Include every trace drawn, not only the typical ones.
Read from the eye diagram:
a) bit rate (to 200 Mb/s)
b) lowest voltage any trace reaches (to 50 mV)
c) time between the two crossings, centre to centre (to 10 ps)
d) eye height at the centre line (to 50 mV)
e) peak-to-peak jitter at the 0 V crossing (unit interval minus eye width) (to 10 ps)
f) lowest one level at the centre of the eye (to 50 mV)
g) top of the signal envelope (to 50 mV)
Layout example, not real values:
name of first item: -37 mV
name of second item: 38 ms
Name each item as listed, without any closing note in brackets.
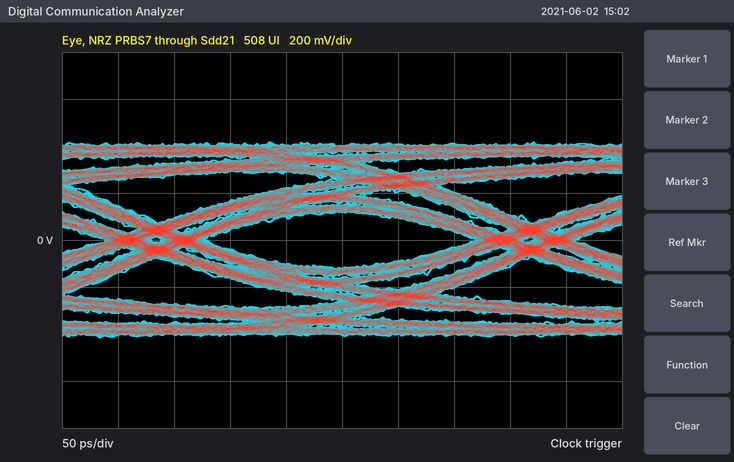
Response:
bit rate: 3.0 Gb/s
lowest voltage any trace reaches: -400 mV
time between the two crossings, centre to centre: 330 ps
eye height at the centre line: 250 mV
peak-to-peak jitter at the 0 V crossing (unit interval minus eye width): 90 ps
lowest one level at the centre of the eye: 100 mV
top of the signal envelope: 400 mV
